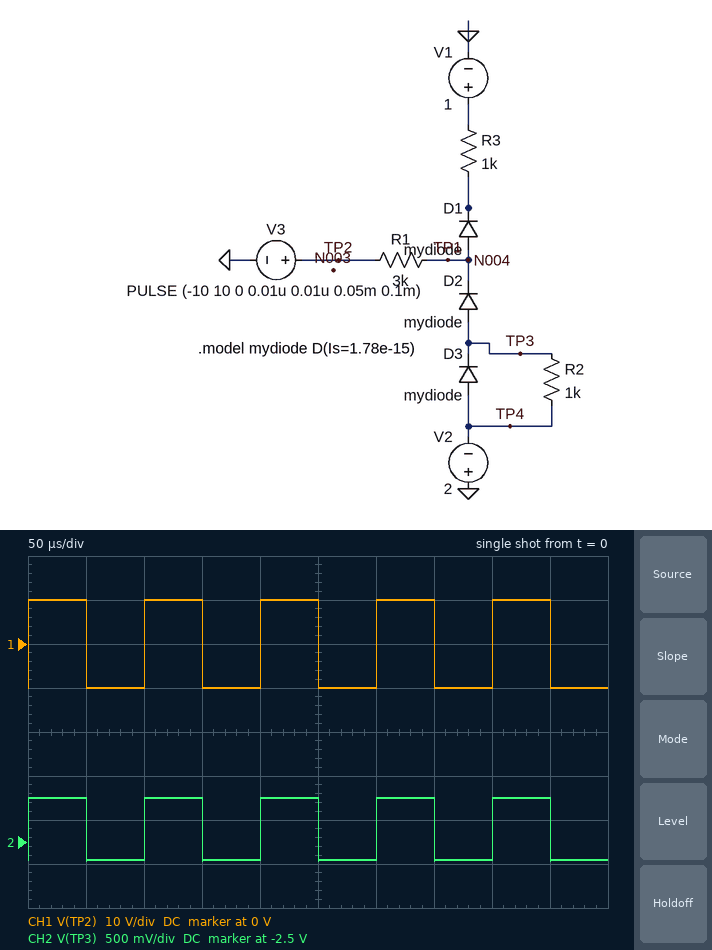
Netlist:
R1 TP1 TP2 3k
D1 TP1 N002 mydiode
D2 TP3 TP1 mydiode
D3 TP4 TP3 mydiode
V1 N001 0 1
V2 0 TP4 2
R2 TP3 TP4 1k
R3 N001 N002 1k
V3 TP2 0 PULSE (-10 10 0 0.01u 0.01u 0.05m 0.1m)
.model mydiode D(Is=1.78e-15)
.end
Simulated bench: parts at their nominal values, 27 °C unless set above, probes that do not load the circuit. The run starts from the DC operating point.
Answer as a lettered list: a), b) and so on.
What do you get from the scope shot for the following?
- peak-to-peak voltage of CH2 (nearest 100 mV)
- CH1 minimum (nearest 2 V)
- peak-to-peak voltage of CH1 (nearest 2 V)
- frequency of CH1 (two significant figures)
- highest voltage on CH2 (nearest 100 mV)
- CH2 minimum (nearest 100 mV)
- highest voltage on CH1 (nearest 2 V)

a) 700 mV
b) -10 V
c) 20 V
d) 10 kHz
e) -2.0 V
f) -2.7 V
g) 10 V
